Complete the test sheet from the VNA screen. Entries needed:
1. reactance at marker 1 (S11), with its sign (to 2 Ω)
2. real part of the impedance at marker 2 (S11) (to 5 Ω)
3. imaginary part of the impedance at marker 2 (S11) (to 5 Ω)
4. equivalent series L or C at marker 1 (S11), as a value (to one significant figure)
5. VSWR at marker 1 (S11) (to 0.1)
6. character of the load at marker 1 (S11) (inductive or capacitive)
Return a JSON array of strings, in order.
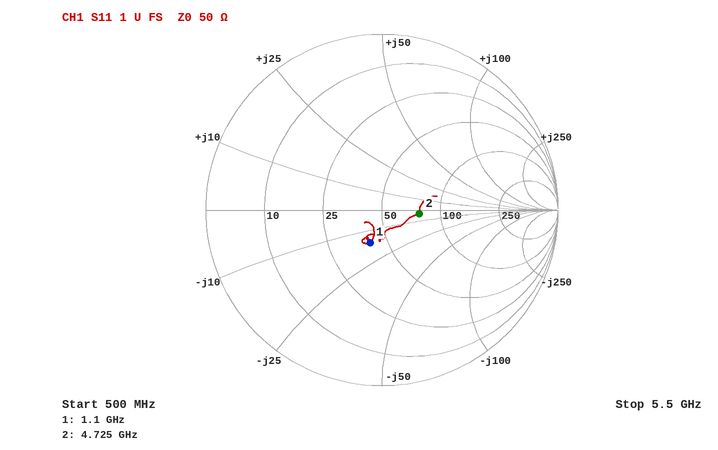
["-16 Ω", "75 Ω", "-5 Ω", "9 pF", "1.5", "capacitive"]
